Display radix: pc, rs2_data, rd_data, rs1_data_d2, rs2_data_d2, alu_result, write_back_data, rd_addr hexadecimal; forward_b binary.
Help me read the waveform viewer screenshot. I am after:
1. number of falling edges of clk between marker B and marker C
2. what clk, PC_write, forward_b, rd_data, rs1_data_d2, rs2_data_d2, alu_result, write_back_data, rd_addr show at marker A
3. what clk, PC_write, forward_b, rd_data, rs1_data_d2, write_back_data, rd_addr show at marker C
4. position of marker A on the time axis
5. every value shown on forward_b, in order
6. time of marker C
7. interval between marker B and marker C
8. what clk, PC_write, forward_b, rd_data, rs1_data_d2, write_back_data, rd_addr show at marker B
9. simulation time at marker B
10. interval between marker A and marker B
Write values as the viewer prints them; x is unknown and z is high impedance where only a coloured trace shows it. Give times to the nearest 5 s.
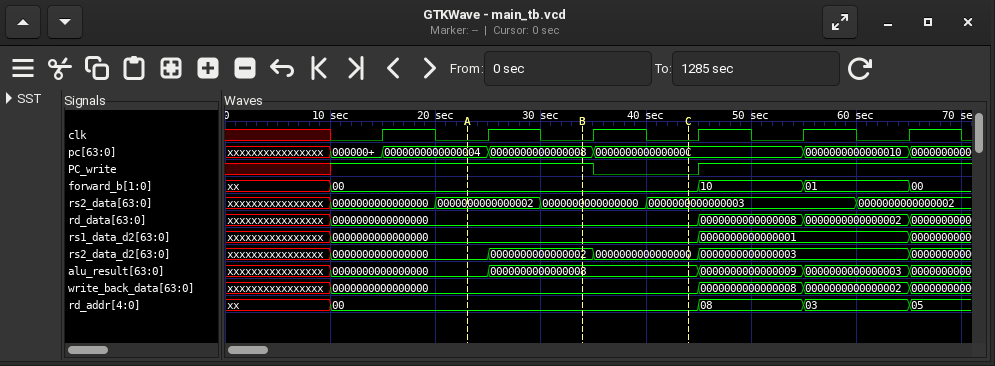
1
clk=0, PC_write=1, forward_b=00, rd_data=0000000000000000, rs1_data_d2=0000000000000000, rs2_data_d2=0000000000000000, alu_result=0000000000000000, write_back_data=0000000000000000, rd_addr=00
clk=0, PC_write=0, forward_b=00, rd_data=0000000000000000, rs1_data_d2=0000000000000000, write_back_data=0000000000000000, rd_addr=00
25 s
xx, 00, 10, 01, 00
45 s
10 s
clk=0, PC_write=1, forward_b=00, rd_data=0000000000000000, rs1_data_d2=0000000000000000, write_back_data=0000000000000000, rd_addr=00
35 s
10 s
